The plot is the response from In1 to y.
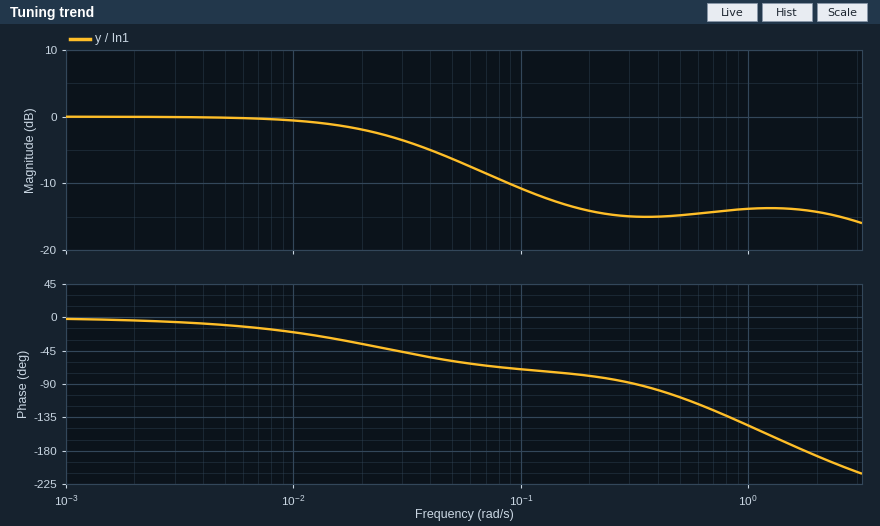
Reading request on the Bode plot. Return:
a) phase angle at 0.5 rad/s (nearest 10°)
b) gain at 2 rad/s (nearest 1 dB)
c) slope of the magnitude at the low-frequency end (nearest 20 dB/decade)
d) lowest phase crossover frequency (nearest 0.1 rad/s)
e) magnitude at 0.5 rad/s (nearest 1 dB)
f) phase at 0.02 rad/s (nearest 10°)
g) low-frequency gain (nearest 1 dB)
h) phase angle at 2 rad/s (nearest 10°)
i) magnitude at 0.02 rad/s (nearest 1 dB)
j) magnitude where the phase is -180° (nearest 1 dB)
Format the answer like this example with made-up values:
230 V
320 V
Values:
-110°
-14 dB
0 dB/decade
1.8 rad/s
-15 dB
-40°
0 dB
-190°
-2 dB
-14 dB
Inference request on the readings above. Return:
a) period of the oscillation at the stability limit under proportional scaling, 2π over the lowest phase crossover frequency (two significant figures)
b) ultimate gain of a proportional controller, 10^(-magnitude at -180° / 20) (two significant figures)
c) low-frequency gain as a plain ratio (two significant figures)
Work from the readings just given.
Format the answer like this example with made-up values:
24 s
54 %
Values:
3.5 s
5.0
1.0
